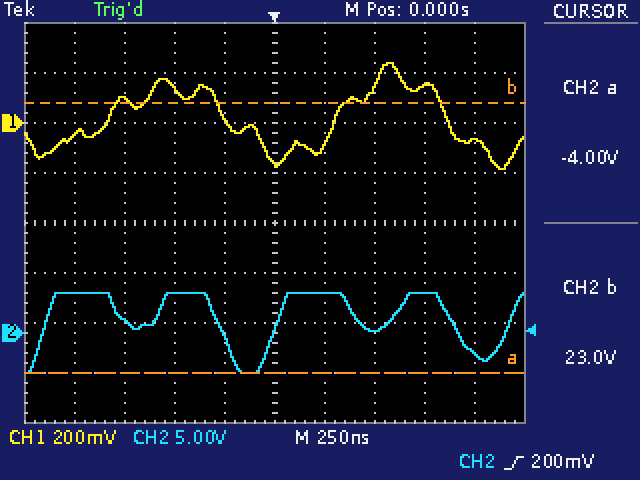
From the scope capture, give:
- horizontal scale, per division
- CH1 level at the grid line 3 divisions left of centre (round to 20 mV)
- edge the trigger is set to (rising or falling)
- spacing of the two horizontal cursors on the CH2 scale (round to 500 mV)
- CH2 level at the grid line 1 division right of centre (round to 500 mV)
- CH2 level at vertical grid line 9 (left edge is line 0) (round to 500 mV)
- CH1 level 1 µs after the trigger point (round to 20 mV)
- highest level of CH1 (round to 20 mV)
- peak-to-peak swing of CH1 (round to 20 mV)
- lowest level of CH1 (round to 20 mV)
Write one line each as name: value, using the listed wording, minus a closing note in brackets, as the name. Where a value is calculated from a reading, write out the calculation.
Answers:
horizontal scale, per division: 250 ns
CH1 level at the grid line 3 divisions left of centre: 100 mV
edge the trigger is set to: rising
spacing of the two horizontal cursors on the CH2 scale: 27.0 V
CH2 level at the grid line 1 division right of centre: 4.0 V
CH2 level at vertical grid line 9 (left edge is line 0): -2.0 V
CH1 level 1 µs after the trigger point: -60 mV
highest level of CH1: 240 mV
peak-to-peak swing of CH1: 240 mV − (-180 mV) = 420 mV
lowest level of CH1: -180 mV
